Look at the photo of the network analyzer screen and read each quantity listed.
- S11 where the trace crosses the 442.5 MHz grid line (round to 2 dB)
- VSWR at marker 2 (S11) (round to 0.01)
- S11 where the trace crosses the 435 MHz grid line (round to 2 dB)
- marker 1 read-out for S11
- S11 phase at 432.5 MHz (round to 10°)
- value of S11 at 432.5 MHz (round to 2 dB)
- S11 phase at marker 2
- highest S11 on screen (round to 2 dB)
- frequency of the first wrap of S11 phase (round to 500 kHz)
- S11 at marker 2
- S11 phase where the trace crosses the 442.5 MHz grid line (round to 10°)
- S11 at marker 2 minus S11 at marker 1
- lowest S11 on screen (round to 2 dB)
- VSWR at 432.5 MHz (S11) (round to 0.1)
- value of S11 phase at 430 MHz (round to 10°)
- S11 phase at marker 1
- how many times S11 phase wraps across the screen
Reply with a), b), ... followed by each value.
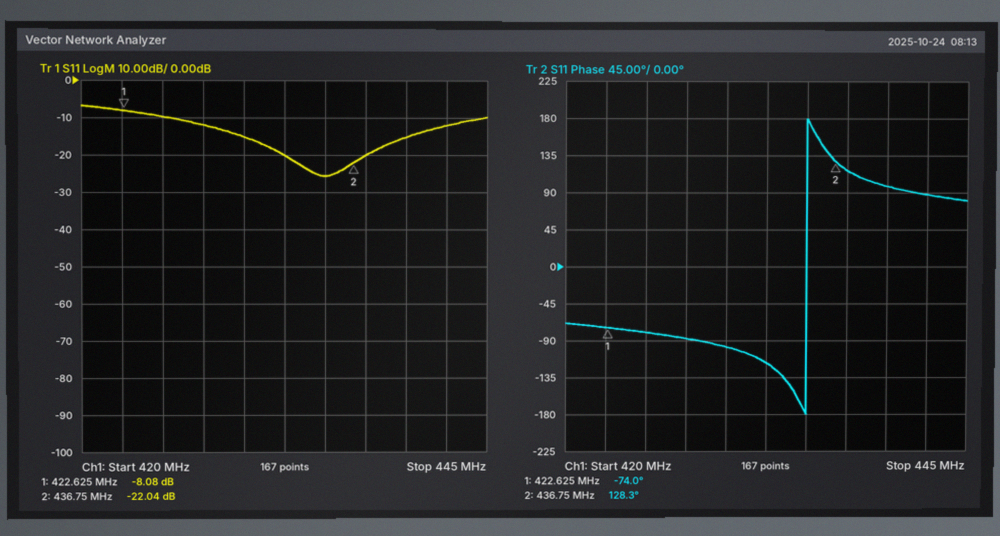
a) -12 dB
b) 1.17
c) -26 dB
d) -8.08 dB
e) -120°
f) -20 dB
g) 128.3°
h) -6 dB
i) 435.0 MHz
j) -22.04 dB
k) 90°
l) -13.96 dB
m) -26 dB
n) 1.2
o) -100°
p) -74.0°
q) 1
